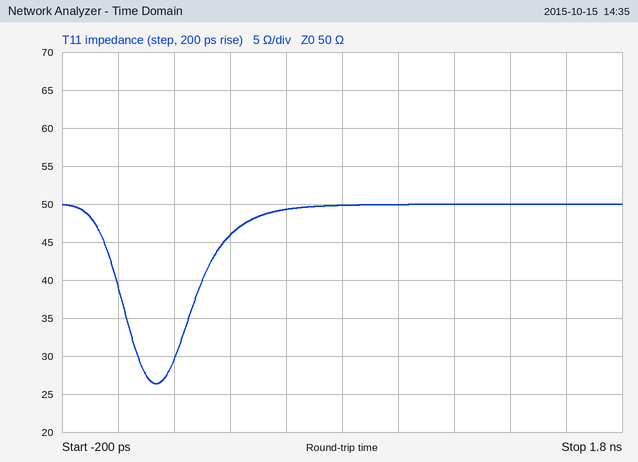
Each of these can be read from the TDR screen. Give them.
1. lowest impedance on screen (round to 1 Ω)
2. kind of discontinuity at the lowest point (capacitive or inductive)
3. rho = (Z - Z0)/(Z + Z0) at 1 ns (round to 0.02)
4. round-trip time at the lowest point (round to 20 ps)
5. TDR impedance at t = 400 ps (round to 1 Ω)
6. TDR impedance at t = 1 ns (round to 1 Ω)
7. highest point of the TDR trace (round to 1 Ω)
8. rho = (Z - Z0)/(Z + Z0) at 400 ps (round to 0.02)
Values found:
26 Ω
capacitive
0.00
140 ps
46 Ω
50 Ω
50 Ω
-0.04
